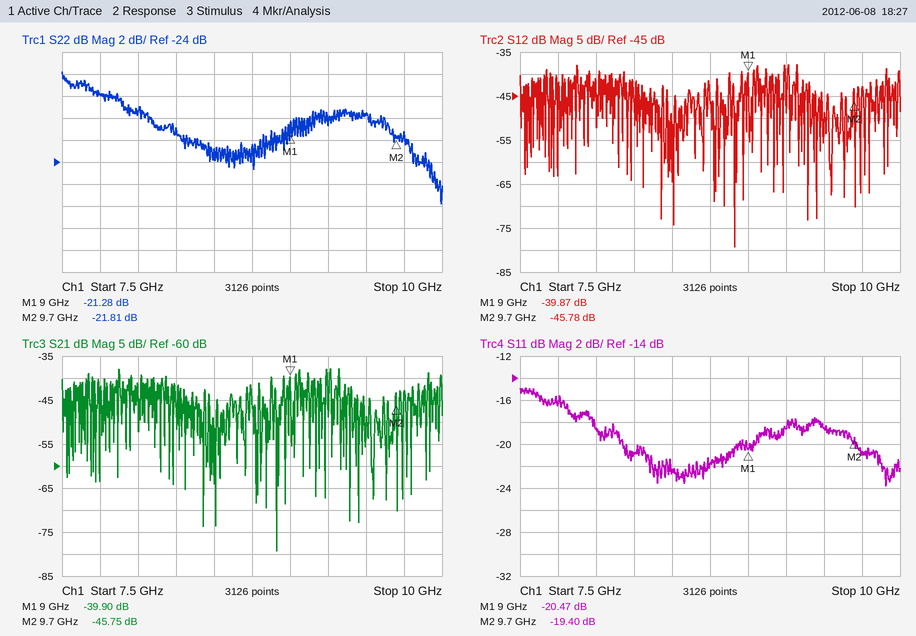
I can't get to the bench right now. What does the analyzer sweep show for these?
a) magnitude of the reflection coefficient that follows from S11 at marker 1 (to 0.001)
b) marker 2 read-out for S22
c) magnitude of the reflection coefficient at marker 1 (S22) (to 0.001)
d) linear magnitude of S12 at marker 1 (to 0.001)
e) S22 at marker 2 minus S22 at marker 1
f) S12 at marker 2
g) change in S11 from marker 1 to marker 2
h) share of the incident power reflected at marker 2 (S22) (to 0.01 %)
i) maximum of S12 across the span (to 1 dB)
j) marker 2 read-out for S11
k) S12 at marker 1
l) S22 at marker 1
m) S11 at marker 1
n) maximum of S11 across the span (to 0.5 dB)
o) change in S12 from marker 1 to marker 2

0.095
-21.81 dB
0.086
0.010
-0.53 dB
-45.78 dB
1.07 dB
0.66 %
-38 dB
-19.40 dB
-39.87 dB
-21.28 dB
-20.47 dB
-15.0 dB
-5.91 dB
